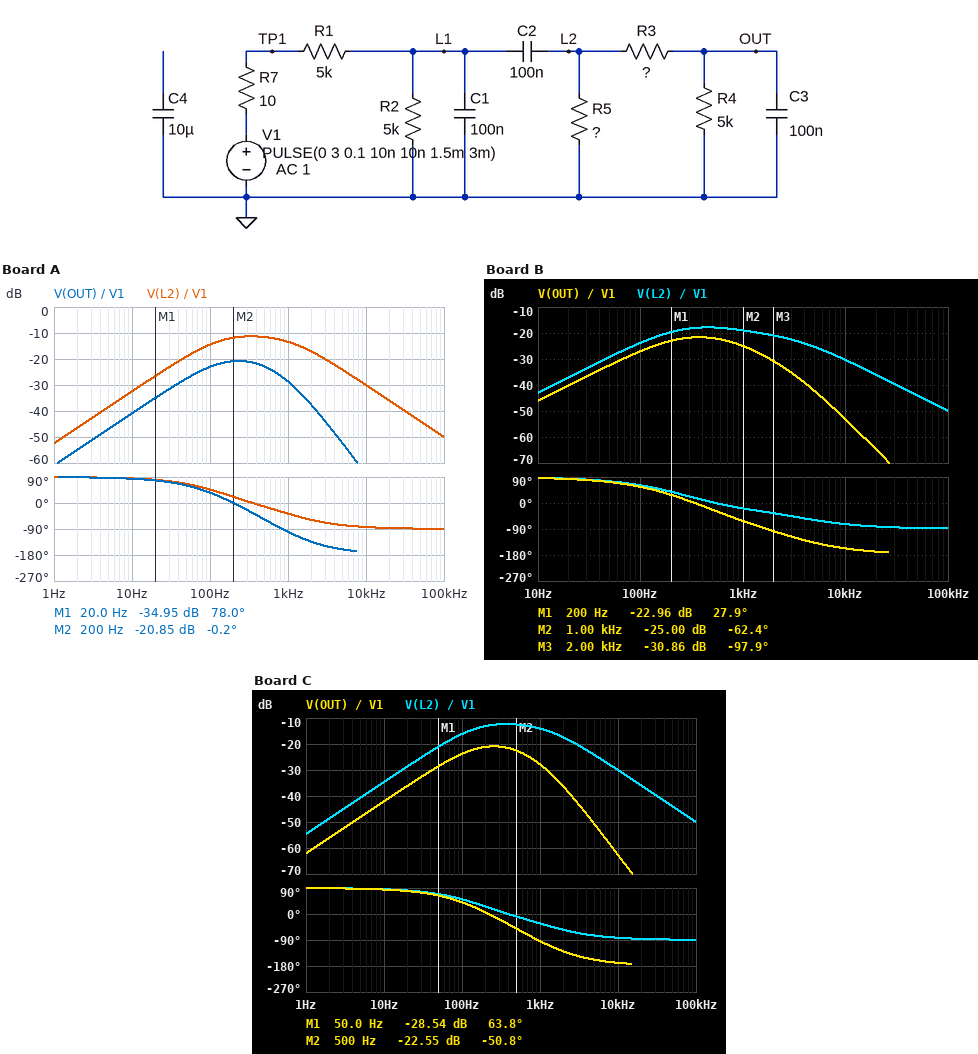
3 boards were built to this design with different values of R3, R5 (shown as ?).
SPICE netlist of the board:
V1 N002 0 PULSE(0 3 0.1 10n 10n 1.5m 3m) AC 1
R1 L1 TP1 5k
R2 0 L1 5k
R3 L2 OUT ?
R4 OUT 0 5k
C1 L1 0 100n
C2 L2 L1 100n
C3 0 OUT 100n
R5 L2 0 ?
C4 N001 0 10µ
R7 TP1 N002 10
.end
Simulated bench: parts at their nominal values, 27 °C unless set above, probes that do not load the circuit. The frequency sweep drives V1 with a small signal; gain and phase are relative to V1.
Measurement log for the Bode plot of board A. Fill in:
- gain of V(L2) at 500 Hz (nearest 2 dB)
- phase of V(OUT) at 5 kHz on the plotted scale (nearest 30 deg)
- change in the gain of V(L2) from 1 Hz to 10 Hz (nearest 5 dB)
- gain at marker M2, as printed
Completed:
-12 dB
-150 deg
20 dB
-20.85 dB
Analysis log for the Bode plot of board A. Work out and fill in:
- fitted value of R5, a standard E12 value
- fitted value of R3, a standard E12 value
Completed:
18 kΩ
8.2 kΩ
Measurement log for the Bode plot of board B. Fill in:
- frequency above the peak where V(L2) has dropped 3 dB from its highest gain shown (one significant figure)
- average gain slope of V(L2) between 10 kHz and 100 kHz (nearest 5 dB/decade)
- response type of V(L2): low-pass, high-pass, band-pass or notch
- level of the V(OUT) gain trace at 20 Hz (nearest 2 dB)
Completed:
2 kHz
-20 dB/decade
band-pass
-40 dB
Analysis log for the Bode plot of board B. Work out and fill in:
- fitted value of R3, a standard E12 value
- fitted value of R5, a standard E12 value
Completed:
2.2 kΩ
3.3 kΩ
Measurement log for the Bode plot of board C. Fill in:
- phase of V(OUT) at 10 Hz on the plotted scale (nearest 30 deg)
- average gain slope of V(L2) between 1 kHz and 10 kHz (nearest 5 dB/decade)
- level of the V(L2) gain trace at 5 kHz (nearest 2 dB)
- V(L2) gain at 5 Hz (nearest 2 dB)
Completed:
90 deg
-15 dB/decade
-24 dB
-40 dB
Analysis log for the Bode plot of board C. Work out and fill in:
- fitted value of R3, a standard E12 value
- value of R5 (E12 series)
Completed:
6.8 kΩ
12 kΩ
